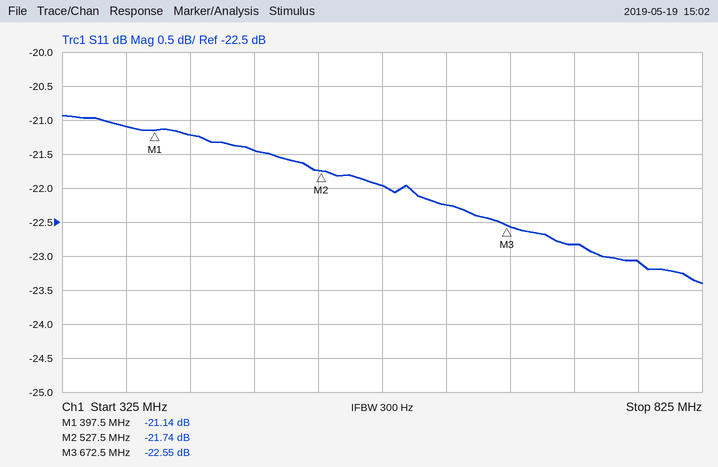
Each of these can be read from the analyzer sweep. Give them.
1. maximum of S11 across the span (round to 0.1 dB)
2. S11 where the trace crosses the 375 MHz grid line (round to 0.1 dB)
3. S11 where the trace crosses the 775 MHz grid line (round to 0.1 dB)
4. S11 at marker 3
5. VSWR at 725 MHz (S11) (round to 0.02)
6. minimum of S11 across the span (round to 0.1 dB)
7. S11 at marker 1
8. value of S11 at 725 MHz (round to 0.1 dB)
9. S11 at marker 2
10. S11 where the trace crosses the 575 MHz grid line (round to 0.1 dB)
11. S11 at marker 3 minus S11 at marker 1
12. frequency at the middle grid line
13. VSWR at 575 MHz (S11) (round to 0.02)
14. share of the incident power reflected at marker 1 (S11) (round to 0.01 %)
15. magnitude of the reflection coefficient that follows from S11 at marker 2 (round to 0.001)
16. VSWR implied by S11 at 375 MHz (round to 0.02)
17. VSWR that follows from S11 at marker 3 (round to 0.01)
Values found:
-20.9 dB
-21.1 dB
-23.1 dB
-22.55 dB
1.16
-23.4 dB
-21.14 dB
-22.8 dB
-21.74 dB
-22.0 dB
-1.41 dB
575 MHz
1.18
0.77 %
0.082
1.20
1.16
